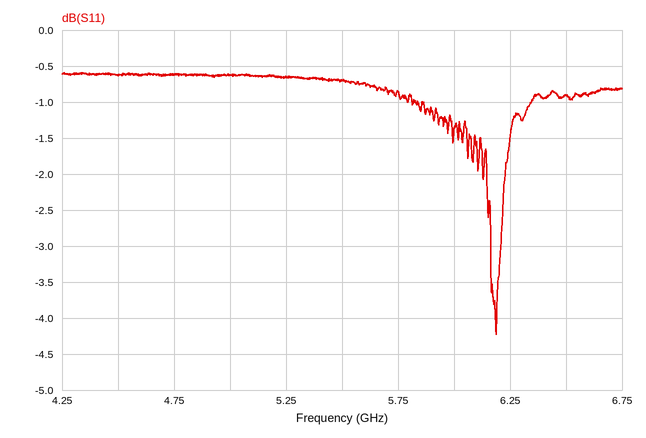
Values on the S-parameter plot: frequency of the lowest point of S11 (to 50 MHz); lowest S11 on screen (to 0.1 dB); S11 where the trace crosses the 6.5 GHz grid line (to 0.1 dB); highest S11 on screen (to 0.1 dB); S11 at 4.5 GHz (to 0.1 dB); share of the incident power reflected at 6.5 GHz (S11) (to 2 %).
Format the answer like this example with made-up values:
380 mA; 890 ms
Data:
6.20 GHz; -4.2 dB; -0.9 dB; -0.6 dB; -0.6 dB; 82 %
